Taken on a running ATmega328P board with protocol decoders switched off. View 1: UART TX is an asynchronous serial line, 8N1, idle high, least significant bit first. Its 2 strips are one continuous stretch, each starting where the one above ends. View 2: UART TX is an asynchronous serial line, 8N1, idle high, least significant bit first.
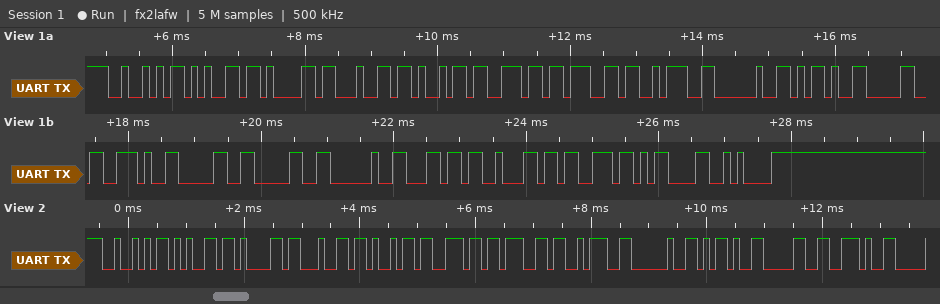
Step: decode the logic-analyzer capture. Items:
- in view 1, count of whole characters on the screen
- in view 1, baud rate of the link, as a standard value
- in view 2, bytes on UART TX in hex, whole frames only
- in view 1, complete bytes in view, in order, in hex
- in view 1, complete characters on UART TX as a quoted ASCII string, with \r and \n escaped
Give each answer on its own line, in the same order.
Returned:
20
9600 baud
52 65 61 64 69 6E 67 3A 20 2D 30 2E
52 65 61 64 69 6E 67 3A 20 2D 30 2E 30 30 20 6C 62 73 0D 0A
"Reading: -0.00 lbs\r\n"
